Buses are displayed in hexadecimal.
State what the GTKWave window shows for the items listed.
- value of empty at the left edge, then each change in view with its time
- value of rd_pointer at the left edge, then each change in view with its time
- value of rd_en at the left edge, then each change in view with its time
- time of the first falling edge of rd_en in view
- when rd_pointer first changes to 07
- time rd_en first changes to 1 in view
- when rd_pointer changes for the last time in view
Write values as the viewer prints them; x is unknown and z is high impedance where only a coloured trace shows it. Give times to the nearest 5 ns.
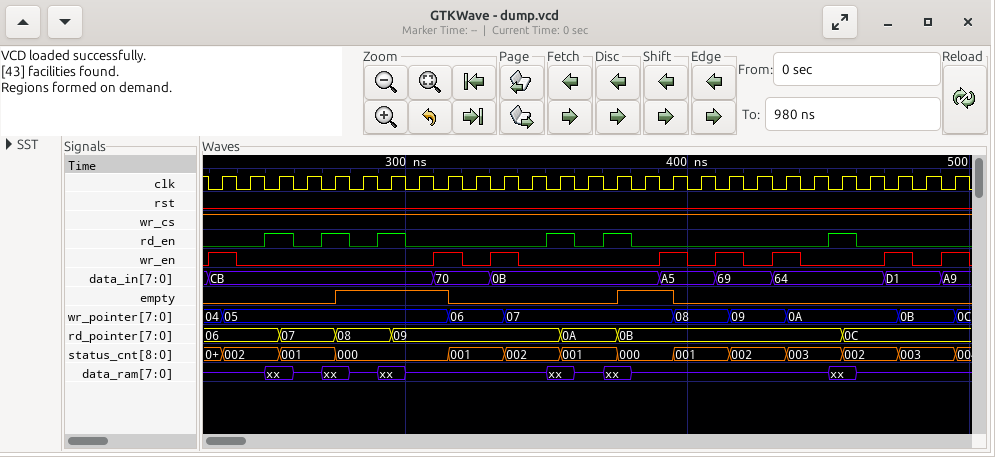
0, 1 at 275 ns, 0 at 315 ns, 1 at 375 ns, 0 at 395 ns
06, 07 at 255 ns, 08 at 275 ns, 09 at 295 ns, 0A at 355 ns, 0B at 375 ns, 0C at 455 ns
0, 1 at 250 ns, 0 at 260 ns, 1 at 270 ns, 0 at 280 ns, 1 at 290 ns, 0 at 300 ns, 1 at 350 ns, 0 at 360 ns, 1 at 370 ns, 0 at 380 ns, 1 at 450 ns, 0 at 460 ns
260 ns
255 ns
250 ns
455 ns
